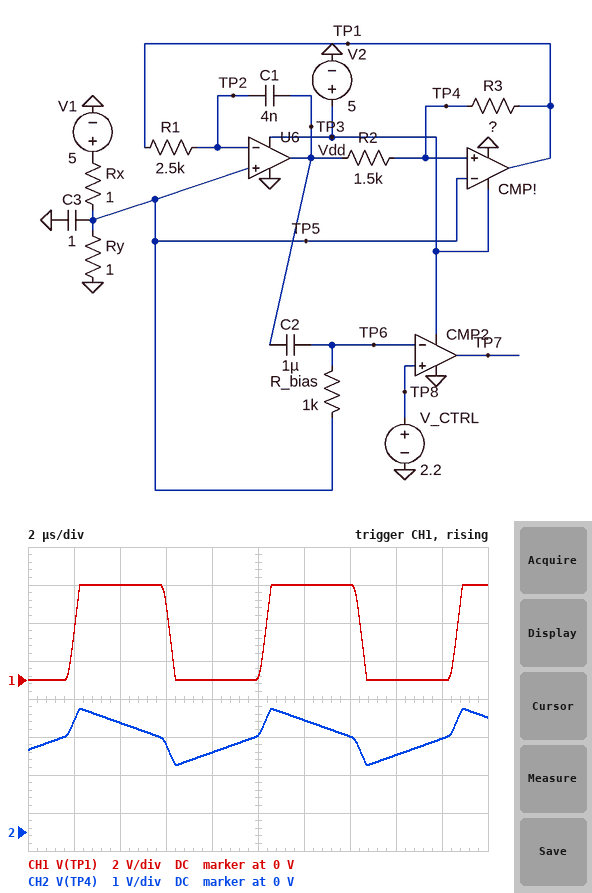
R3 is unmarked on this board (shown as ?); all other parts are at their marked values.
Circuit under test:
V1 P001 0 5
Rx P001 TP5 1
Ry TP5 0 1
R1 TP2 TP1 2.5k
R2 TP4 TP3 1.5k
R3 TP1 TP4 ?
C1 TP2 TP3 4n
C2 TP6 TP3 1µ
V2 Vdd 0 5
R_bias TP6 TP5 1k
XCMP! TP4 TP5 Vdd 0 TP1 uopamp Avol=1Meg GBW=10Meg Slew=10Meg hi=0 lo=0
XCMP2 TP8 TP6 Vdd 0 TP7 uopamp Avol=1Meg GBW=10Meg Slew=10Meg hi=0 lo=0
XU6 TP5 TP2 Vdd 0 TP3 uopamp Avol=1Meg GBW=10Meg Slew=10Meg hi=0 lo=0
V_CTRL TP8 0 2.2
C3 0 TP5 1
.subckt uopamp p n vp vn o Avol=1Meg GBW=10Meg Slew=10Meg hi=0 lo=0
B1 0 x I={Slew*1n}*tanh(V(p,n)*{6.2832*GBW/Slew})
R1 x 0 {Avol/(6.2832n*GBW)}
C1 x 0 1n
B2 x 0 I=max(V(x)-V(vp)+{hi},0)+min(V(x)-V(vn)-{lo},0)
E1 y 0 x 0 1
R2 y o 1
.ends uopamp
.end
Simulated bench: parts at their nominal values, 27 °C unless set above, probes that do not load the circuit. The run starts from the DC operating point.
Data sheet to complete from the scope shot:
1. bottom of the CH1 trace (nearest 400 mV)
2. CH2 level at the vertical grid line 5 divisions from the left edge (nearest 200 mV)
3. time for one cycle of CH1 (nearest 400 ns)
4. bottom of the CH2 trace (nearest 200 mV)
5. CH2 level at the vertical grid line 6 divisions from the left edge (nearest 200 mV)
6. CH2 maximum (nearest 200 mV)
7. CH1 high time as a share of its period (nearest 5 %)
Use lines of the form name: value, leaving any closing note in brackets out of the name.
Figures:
bottom of the CH1 trace: 0 V
CH2 level at the vertical grid line 5 divisions from the left edge: 2.6 V
time for one cycle of CH1: 8.4 µs
bottom of the CH2 trace: 1.8 V
CH2 level at the vertical grid line 6 divisions from the left edge: 3.0 V
CH2 maximum: 3.2 V
CH1 high time as a share of its period: 50 %
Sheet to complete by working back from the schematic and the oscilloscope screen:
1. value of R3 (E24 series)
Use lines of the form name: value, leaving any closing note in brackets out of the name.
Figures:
value of R3: 9.1 kΩ
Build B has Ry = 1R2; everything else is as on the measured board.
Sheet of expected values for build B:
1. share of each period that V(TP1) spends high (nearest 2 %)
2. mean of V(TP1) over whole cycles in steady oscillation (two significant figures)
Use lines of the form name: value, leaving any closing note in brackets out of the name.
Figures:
share of each period that V(TP1) spends high: 54 %
mean of V(TP1) over whole cycles in steady oscillation: 2.7 V
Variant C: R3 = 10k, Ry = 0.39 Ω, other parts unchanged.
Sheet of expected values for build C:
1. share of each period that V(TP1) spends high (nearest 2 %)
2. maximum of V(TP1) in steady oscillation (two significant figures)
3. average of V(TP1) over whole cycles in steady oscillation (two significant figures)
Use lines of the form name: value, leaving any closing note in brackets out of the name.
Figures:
share of each period that V(TP1) spends high: 28 %
maximum of V(TP1) in steady oscillation: 5.0 V
average of V(TP1) over whole cycles in steady oscillation: 1.4 V
